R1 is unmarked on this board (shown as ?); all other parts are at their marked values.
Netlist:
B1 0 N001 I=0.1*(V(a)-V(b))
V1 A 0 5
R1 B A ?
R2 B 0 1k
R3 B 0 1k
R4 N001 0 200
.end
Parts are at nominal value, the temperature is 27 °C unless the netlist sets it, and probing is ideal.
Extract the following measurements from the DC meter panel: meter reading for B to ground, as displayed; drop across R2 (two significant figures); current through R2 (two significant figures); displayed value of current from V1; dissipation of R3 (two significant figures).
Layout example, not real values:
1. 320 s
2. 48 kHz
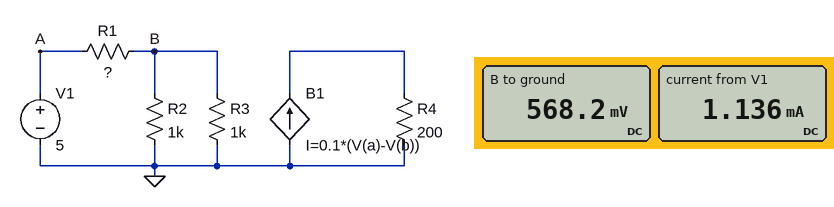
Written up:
1. 568.2 mV
2. 570 mV
3. 570 µA
4. 1.136 mA
5. 320 µW
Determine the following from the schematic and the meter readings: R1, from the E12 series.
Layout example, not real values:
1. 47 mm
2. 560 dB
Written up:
1. 3.9 kΩ
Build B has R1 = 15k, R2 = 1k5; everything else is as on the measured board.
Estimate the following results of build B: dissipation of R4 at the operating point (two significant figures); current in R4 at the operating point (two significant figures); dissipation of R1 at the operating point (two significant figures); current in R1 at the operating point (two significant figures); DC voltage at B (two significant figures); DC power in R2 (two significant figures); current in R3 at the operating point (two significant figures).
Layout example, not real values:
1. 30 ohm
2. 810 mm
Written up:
1. 46 W
2. 480 mA
3. 1.5 mW
4. 320 µA
5. 190 mV
6. 25 µW
7. 190 µA
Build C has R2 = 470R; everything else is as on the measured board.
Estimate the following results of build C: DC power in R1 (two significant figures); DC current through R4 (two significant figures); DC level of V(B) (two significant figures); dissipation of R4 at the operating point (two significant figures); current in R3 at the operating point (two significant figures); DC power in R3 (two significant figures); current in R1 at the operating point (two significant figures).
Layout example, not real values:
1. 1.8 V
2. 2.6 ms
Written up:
1. 5.5 mW
2. 460 mA
3. 380 mV
4. 43 W
5. 380 µA
6. 140 µW
7. 1.2 mA
